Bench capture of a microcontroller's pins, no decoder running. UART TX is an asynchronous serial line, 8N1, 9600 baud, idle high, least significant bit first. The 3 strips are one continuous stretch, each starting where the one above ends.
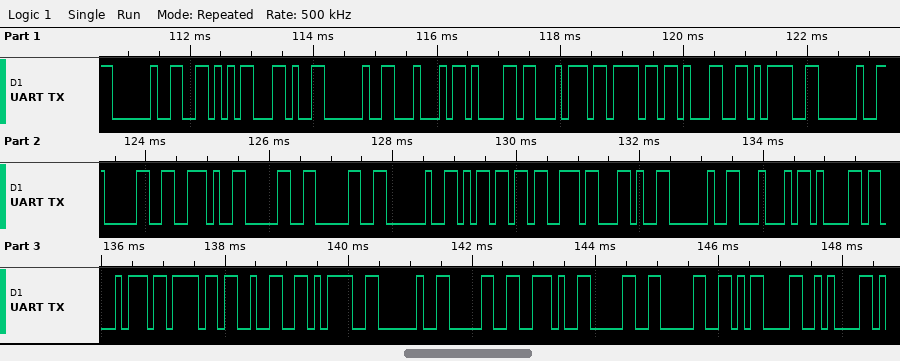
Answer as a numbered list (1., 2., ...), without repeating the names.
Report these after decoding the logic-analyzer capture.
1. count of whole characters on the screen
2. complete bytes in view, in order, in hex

1. 33
2. 20 56 2C 20 44 61 74 6F 31 3D 20 30 2E 30 30 20 6D 73 2C 20 44 61 74 6F 32 3D 20 30 2E 30 30 0D 0A
